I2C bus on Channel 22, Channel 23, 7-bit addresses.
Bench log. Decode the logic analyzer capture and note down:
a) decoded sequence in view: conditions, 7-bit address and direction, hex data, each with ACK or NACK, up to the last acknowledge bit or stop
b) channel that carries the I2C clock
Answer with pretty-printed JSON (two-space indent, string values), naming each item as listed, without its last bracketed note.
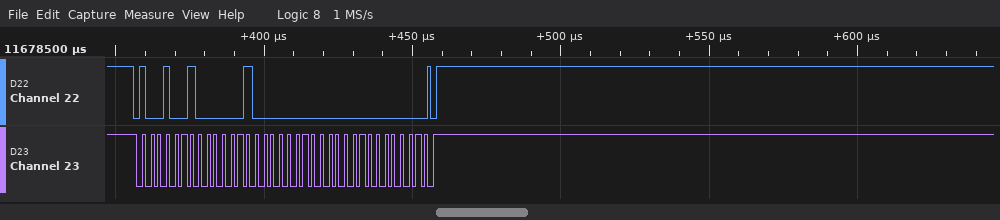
{
  "decoded sequence in view: conditions, 7-bit address and direction, hex data, each with ACK or NACK, up to the last acknowledge bit or stop": "start, address 49 write ACK, 08 ACK, 00 ACK, 00 ACK, stop",
  "channel that carries the I2C clock": "Channel 23"
}
